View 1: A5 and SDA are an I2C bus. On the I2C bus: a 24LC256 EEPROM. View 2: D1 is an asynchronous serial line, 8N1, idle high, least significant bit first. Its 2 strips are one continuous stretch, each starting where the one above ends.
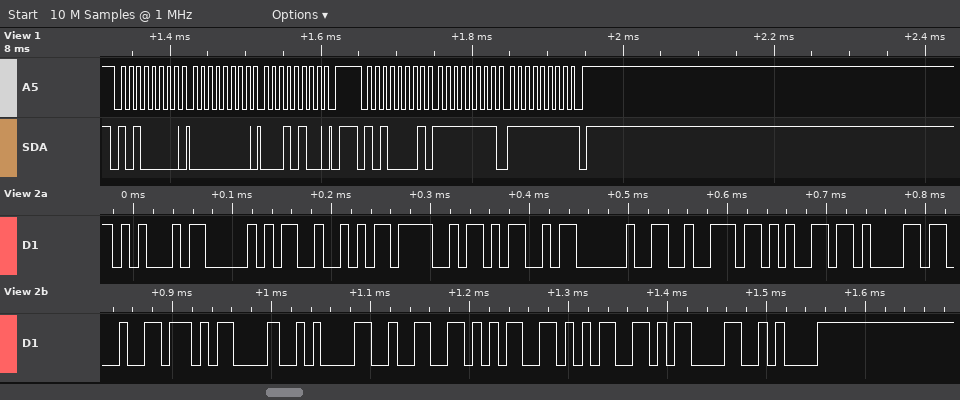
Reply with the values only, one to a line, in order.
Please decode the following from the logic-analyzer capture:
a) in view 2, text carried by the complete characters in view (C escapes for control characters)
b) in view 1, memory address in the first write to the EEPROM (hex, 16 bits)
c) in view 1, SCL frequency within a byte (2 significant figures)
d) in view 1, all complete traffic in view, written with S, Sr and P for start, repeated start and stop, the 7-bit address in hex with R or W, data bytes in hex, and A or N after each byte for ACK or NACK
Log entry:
"EPROM read\r\n255\r\n"
0x0014
100 kHz
S 50W A 00 A 14 A P S 50R A FF A FF N P
